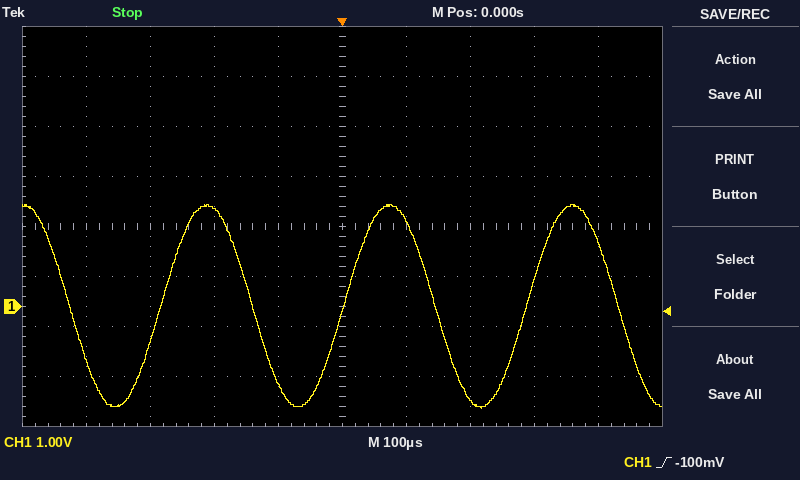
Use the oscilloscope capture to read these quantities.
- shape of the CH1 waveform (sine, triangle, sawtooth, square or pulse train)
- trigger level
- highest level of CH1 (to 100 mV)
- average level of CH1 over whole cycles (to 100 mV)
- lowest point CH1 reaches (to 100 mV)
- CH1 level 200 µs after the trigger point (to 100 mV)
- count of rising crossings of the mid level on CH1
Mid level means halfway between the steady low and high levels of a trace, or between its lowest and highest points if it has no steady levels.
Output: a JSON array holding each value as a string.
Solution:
["sine", "-100 mV", "2.0 V", "0.0 V", "-2.0 V", "-1.9 V", "3"]
